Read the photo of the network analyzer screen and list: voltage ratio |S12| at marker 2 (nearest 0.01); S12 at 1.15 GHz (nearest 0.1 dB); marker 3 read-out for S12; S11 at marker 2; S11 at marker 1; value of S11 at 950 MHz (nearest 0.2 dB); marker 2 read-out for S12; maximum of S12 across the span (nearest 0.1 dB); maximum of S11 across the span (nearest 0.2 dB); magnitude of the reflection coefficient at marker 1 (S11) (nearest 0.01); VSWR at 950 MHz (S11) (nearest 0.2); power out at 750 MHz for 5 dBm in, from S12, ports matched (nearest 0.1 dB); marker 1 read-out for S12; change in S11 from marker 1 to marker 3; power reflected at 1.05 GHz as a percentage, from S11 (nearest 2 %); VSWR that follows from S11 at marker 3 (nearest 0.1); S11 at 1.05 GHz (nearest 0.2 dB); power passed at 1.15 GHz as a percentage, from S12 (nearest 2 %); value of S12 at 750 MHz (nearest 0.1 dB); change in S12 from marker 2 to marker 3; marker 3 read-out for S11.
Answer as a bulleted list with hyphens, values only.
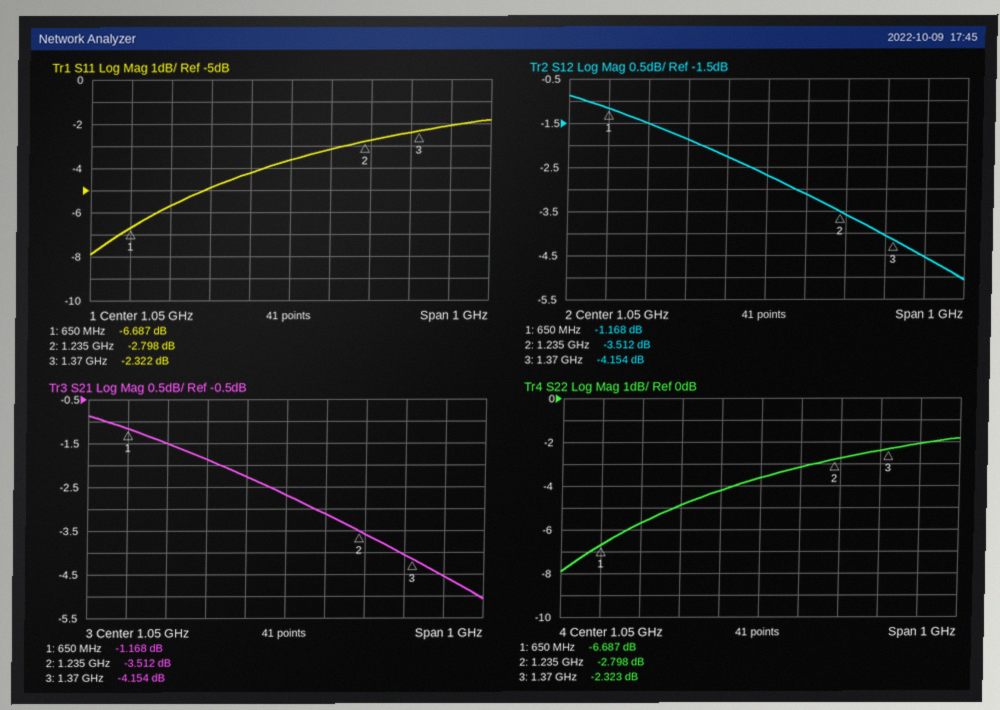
- 0.67
- -3.1 dB
- -4.154 dB
- -2.798 dB
- -6.687 dB
- -4.2 dB
- -3.512 dB
- -0.9 dB
- -1.8 dB
- 0.46
- 4.2
- 3.5 dBm
- -1.168 dB
- 4.365 dB
- 44 %
- 7.5
- -3.6 dB
- 48 %
- -1.5 dB
- -0.642 dB
- -2.322 dB
